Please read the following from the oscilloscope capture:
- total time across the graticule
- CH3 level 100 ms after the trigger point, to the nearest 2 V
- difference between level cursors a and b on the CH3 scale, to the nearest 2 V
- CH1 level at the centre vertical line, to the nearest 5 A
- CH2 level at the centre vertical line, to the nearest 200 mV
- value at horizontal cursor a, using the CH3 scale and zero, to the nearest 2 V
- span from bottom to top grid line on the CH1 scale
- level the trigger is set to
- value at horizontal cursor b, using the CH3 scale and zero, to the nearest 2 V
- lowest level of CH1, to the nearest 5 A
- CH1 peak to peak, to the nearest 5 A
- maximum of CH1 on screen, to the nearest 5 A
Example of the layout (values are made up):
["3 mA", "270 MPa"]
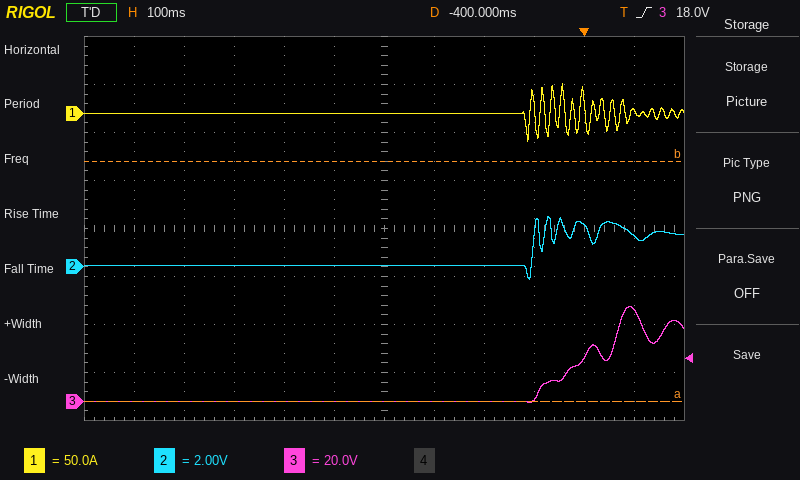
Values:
["1.2 s", "38 V", "100 V", "0 A", "0.0 V", "0 V", "400 A", "18.0 V", "100 V", "-30 A", "60 A", "30 A"]
